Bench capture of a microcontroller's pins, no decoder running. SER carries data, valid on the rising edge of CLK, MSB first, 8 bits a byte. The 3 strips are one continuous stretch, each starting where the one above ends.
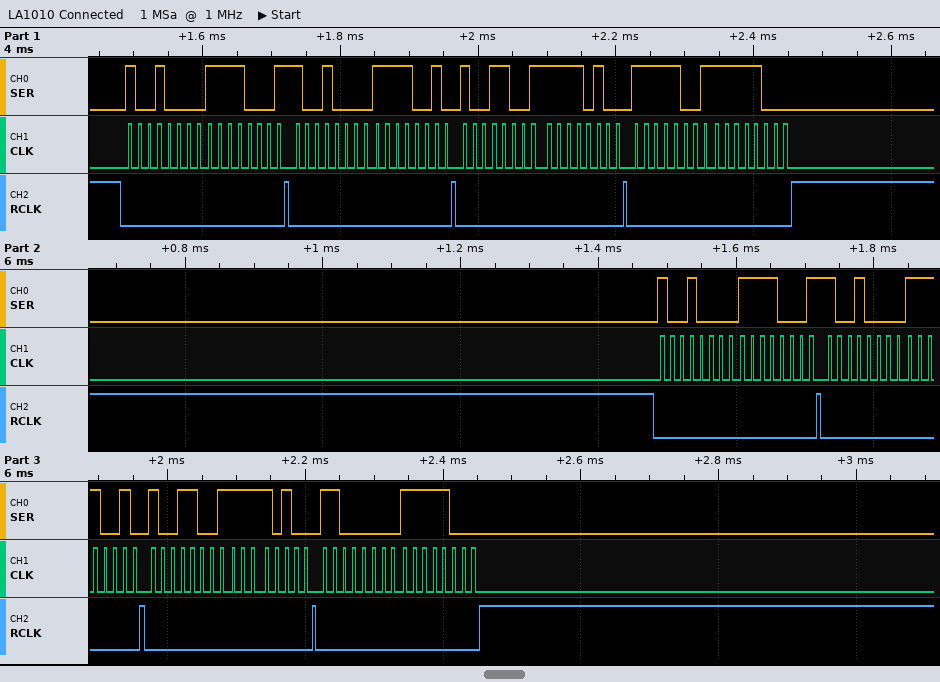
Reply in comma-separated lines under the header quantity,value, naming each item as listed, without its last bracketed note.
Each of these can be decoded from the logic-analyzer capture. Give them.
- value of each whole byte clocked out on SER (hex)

quantity,value
value of each whole byte clocked out on SER,90 F1 90 F2 99 F4 F9 F8 90 F1 90 F2 99 F4 C0 F8
